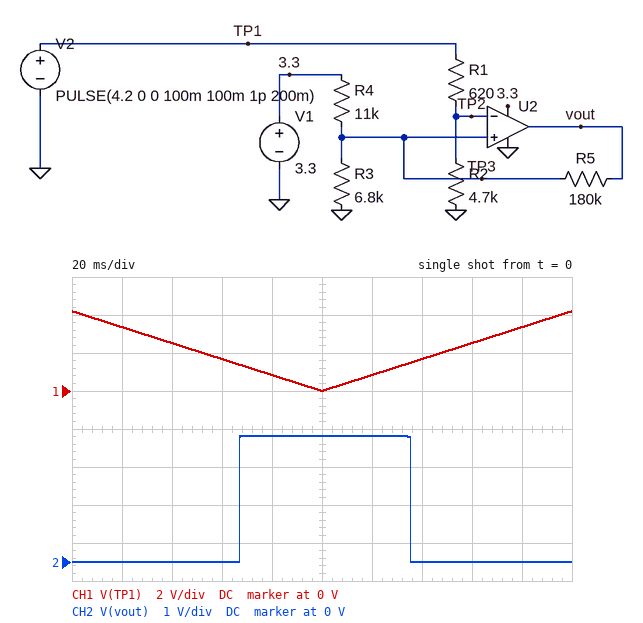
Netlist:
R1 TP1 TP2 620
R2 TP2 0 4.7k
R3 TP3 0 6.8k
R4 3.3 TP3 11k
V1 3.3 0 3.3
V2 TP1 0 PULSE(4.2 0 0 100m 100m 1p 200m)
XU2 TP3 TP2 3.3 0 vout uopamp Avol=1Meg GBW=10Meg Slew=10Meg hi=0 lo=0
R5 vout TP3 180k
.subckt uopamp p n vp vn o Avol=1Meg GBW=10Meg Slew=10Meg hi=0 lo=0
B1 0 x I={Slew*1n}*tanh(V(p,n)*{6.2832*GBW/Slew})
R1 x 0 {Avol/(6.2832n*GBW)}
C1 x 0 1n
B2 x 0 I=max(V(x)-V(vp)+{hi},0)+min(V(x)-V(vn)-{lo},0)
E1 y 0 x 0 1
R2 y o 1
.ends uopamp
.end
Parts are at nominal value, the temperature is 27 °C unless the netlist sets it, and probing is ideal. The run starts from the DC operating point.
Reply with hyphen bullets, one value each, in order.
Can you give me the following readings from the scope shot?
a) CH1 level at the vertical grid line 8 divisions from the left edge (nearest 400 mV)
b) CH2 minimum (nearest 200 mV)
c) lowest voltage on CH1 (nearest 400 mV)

- 2.4 V
- 0 V
- 0 V
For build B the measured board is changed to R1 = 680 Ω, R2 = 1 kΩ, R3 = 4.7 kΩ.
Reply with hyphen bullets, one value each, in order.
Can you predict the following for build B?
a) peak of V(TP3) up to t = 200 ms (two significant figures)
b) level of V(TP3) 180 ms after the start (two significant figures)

- 1.0 V
- 970 mV
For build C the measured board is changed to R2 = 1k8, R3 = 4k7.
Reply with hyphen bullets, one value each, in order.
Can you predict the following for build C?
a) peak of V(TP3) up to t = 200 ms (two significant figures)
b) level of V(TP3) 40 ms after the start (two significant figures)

- 1.0 V
- 970 mV
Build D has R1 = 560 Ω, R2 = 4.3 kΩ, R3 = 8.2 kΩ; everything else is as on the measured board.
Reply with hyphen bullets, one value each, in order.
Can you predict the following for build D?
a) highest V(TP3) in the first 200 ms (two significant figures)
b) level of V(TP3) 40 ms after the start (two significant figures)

- 1.5 V
- 1.4 V
